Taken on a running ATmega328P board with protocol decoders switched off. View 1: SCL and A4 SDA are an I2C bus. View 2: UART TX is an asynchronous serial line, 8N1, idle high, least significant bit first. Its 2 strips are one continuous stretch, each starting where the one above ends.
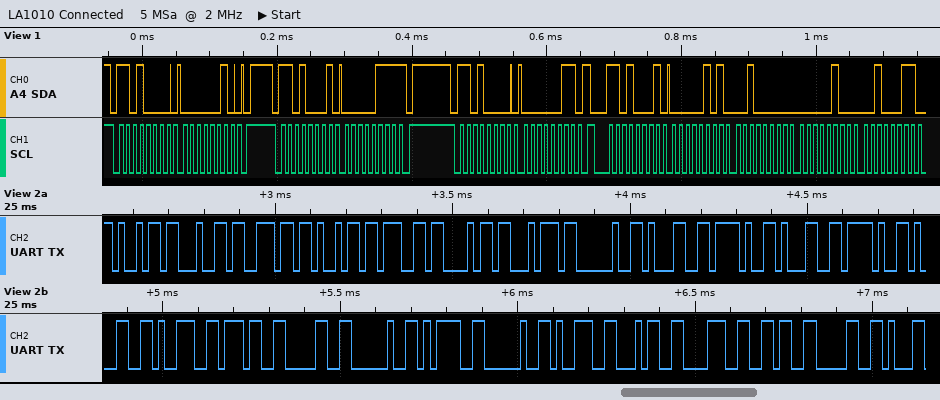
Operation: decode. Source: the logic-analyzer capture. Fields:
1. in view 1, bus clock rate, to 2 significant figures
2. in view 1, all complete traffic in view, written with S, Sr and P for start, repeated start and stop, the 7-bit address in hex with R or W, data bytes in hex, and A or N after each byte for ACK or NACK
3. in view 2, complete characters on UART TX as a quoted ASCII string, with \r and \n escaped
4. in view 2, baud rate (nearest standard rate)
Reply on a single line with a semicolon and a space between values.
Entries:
100 kHz; S 68W A 02 A P S 68R A 07 N P S 68W A 03 A Sr 68R A 05 A 20 A 04 A 23 A; "idnight 1/1/1970 = 94860"; 57600 baud
